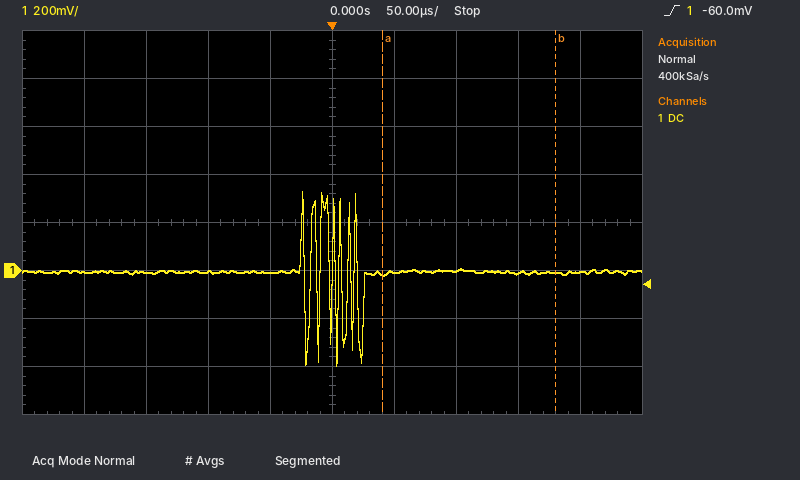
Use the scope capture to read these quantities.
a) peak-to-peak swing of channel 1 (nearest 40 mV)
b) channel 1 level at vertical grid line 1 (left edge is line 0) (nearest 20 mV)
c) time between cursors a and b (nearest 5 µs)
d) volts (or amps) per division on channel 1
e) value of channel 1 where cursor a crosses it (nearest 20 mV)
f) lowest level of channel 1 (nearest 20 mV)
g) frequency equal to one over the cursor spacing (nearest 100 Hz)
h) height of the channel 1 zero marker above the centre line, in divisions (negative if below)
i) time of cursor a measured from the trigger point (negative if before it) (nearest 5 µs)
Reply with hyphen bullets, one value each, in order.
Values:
- 720 mV
- 0 mV
- 140 µs
- 200 mV
- -20 mV
- -400 mV
- 7.1 kHz
- -1.0 div
- +40 µs
